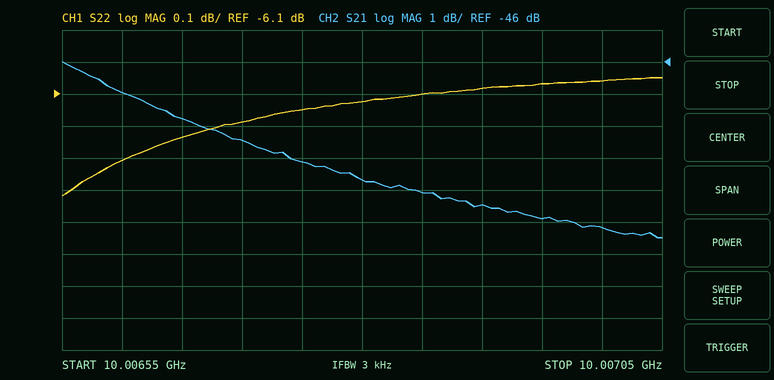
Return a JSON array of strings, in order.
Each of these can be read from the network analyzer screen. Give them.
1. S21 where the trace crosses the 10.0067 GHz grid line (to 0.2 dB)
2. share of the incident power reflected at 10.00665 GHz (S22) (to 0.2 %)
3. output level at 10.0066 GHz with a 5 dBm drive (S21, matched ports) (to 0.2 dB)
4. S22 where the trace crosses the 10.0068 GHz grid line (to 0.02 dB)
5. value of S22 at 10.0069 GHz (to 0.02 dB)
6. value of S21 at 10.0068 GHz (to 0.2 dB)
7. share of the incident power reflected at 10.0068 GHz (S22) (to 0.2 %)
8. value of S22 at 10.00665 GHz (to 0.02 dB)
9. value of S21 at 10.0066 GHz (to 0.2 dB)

["-48.4 dB", "23.8 %", "-42.0 dBm", "-6.12 dB", "-6.08 dB", "-49.6 dB", "24.4 %", "-6.24 dB", "-47.0 dB"]
